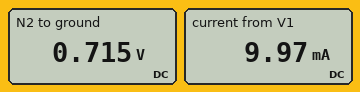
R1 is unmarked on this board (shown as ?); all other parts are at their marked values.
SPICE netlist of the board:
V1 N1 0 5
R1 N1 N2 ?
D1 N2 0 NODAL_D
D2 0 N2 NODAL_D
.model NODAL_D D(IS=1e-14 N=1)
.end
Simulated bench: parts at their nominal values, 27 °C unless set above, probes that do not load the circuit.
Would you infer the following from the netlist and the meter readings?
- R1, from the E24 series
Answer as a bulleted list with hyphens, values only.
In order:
- 430 Ω
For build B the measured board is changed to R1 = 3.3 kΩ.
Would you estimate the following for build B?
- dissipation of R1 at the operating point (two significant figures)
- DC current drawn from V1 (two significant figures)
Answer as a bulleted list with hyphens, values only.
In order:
- 5.7 mW
- 1.3 mA
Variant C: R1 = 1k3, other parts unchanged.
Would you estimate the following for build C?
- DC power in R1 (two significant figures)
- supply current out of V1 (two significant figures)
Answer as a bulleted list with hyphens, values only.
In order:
- 14 mW
- 3.3 mA
